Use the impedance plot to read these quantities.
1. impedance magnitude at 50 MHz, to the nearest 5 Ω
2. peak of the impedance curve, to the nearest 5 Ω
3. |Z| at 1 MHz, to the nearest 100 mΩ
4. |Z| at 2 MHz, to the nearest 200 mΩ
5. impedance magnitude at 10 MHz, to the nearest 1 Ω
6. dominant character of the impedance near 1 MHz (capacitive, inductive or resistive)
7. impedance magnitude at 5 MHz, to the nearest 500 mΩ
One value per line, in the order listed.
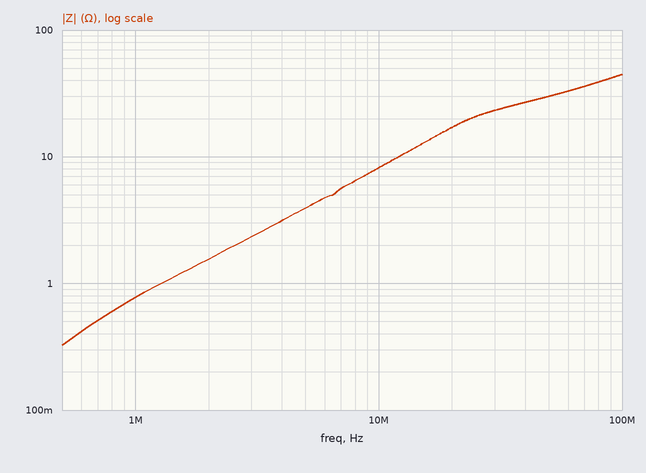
30 Ω
45 Ω
800 mΩ
1.6 Ω
8 Ω
inductive
4.0 Ω
